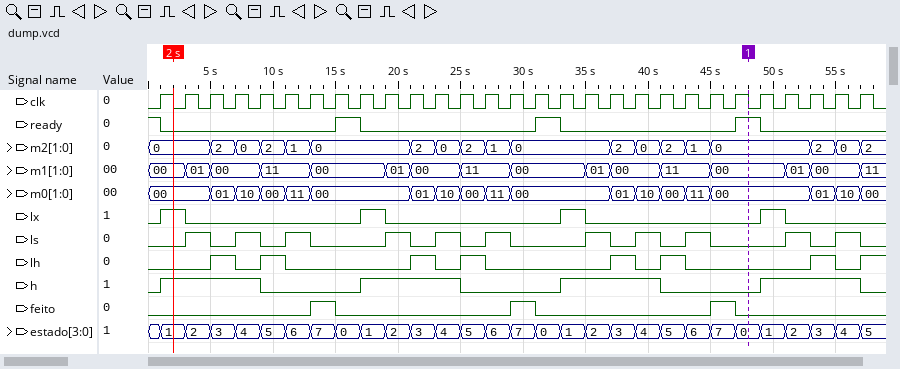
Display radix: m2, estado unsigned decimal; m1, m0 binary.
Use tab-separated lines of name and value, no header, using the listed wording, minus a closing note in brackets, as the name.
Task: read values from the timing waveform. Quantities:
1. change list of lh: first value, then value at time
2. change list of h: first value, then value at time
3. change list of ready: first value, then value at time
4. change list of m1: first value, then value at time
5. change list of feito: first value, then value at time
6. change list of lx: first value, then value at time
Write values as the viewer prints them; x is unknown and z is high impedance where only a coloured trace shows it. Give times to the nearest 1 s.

change list of lh: first value, then value at time	0, 1 at 5 s, 0 at 7 s, 1 at 9 s, 0 at 11 s, 1 at 21 s, 0 at 23 s, 1 at 25 s, 0 at 27 s, 1 at 37 s, 0 at 39 s, 1 at 41 s, 0 at 43 s, 1 at 53 s, 0 at 55 s, 1 at 57 s
change list of h: first value, then value at time	0, 1 at 1 s, 0 at 9 s, 1 at 17 s, 0 at 25 s, 1 at 33 s, 0 at 41 s, 1 at 49 s, 0 at 57 s
change list of ready: first value, then value at time	1, 0 at 1 s, 1 at 15 s, 0 at 17 s, 1 at 31 s, 0 at 33 s, 1 at 47 s, 0 at 49 s
change list of m1: first value, then value at time	00, 01 at 3 s, 00 at 5 s, 11 at 9 s, 00 at 13 s, 01 at 19 s, 00 at 21 s, 11 at 25 s, 00 at 29 s, 01 at 35 s, 00 at 37 s, 11 at 41 s, 00 at 45 s, 01 at 51 s, 00 at 53 s, 11 at 57 s
change list of feito: first value, then value at time	0, 1 at 13 s, 0 at 15 s, 1 at 29 s, 0 at 31 s, 1 at 45 s, 0 at 47 s
change list of lx: first value, then value at time	0, 1 at 1 s, 0 at 3 s, 1 at 17 s, 0 at 19 s, 1 at 33 s, 0 at 35 s, 1 at 49 s, 0 at 51 s
